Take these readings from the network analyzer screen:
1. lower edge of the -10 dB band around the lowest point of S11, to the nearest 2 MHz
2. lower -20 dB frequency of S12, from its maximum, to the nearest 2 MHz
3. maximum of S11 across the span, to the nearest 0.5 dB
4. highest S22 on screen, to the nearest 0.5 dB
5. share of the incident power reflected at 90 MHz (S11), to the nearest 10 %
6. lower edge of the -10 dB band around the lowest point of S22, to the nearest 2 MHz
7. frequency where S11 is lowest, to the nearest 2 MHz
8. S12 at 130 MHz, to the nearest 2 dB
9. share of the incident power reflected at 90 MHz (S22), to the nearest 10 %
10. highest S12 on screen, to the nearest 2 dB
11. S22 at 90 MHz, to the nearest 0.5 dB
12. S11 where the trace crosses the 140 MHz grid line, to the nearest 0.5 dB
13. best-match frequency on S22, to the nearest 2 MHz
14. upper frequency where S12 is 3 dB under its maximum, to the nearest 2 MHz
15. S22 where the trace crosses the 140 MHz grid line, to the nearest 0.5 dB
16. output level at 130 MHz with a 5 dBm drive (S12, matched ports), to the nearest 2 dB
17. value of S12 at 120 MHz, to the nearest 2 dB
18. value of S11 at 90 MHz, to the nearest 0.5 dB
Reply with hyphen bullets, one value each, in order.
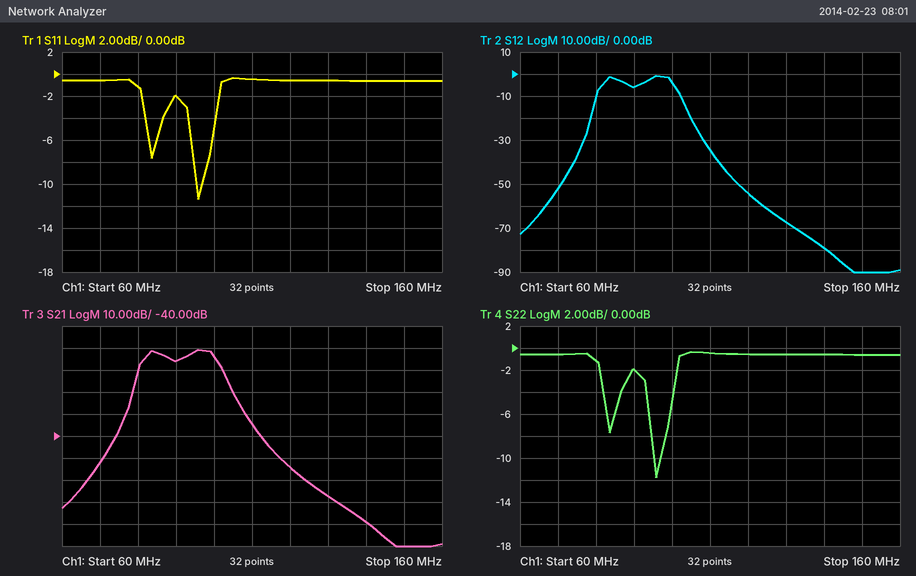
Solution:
- 96 MHz
- 78 MHz
- -0.5 dB
- -0.5 dB
- 60 %
- 96 MHz
- 96 MHz
- -68 dB
- 60 %
- 0 dB
- -2.0 dB
- -0.5 dB
- 96 MHz
- 100 MHz
- -0.5 dB
- -62 dBm
- -54 dB
- -2.0 dB
